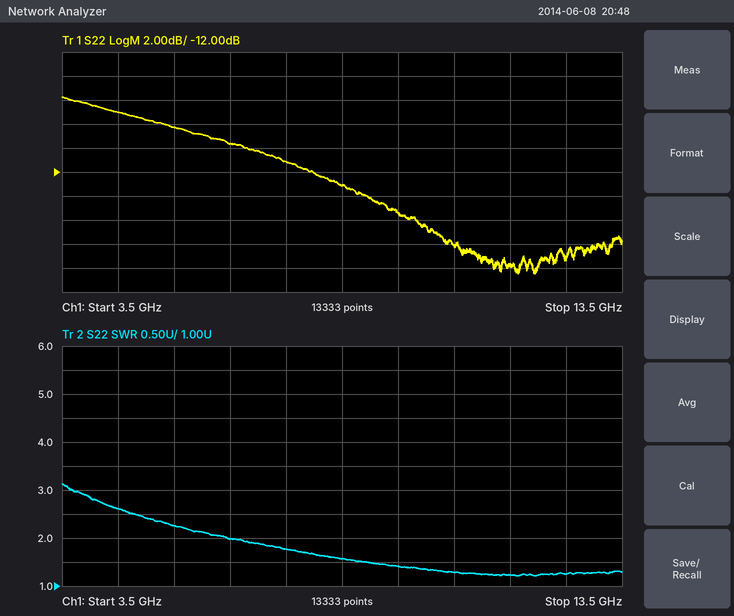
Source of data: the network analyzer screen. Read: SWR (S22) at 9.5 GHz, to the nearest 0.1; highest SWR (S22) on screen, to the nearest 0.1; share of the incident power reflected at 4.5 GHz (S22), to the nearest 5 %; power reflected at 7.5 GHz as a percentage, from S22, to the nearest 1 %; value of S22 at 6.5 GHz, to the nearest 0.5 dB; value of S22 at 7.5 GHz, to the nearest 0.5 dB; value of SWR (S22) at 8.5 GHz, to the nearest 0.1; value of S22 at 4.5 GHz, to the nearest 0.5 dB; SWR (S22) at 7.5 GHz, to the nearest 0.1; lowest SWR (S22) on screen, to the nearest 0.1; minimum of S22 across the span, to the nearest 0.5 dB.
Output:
1.4
3.1
20 %
8 %
-9.5 dB
-11.0 dB
1.6
-7.0 dB
1.8
1.2
-20.5 dB
